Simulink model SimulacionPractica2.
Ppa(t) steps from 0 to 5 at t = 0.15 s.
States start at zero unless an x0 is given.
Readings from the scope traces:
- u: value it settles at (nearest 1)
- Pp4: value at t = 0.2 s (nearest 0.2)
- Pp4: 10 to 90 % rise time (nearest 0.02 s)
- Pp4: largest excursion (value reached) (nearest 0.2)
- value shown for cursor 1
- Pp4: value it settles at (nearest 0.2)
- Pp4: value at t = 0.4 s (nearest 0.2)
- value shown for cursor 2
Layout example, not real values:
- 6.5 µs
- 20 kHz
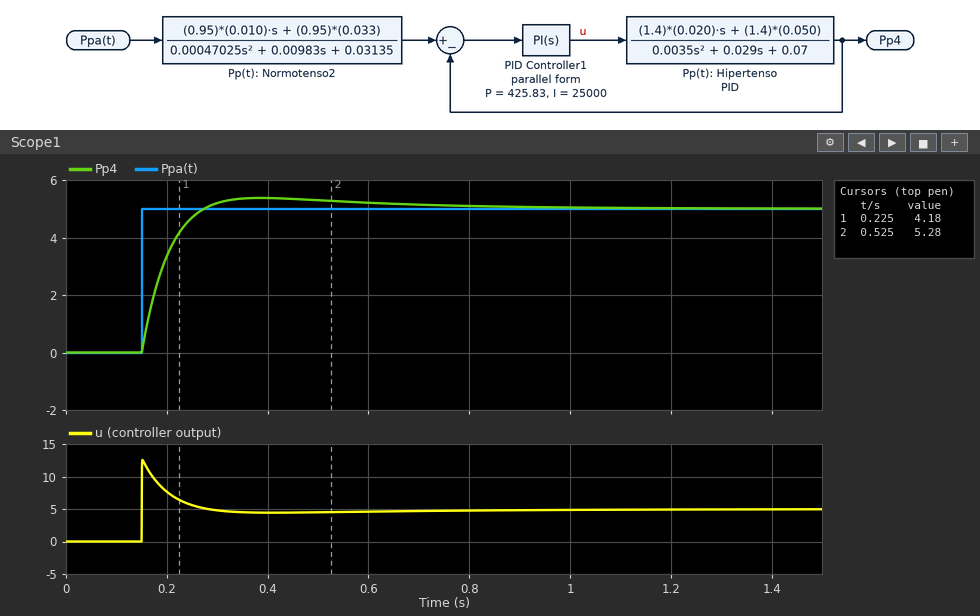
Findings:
- 5
- 3.4
- 0.08 s
- 5.4
- 4.18
- 5.0
- 5.4
- 5.28
